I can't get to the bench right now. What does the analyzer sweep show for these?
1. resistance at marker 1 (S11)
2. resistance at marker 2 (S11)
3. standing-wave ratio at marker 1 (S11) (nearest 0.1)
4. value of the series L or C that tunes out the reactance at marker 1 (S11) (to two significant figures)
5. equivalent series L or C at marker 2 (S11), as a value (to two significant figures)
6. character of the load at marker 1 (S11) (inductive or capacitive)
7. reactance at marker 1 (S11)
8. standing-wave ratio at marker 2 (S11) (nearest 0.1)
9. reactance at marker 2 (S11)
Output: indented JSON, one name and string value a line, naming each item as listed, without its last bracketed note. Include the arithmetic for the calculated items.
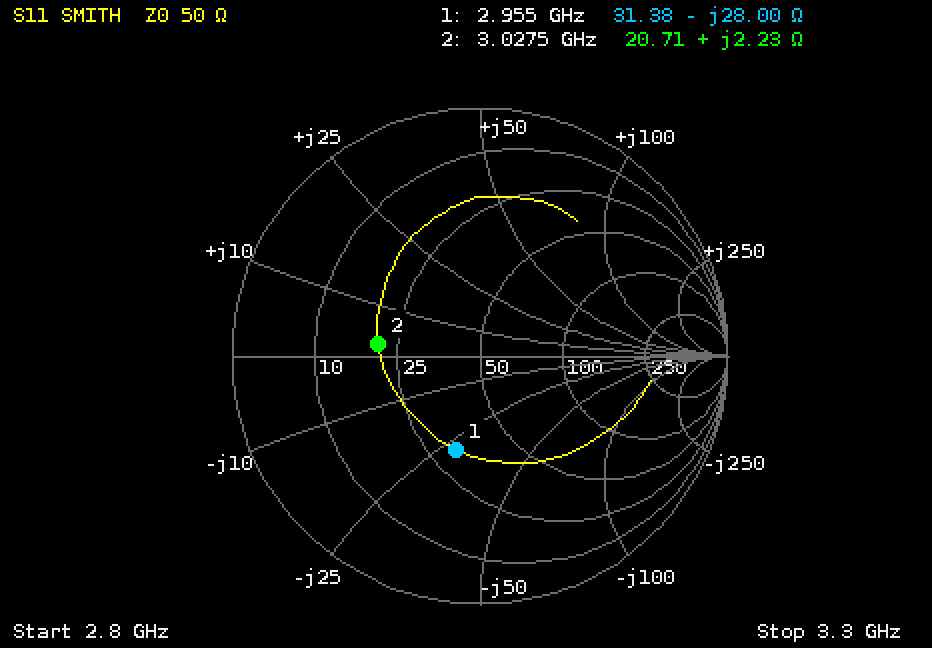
{
  "resistance at marker 1": "31.38 Ω",
  "resistance at marker 2": "20.71 Ω",
  "standing-wave ratio at marker 1 (S11)": "2.3",
  "value of the series L or C that tunes out the reactance at marker 1 (S11)": "L = 28 Ω/(2π × 2.955 GHz) ≈ 1.5 nH",
  "equivalent series L or C at marker 2 (S11), as a value": "L = 2.23 Ω/(2π × 3.0275 GHz) ≈ 117 pH, so 120 pH to two significant figures",
  "character of the load at marker 1 (S11)": "capacitive",
  "reactance at marker 1": "-28.00 Ω",
  "standing-wave ratio at marker 2 (S11)": "2.4",
  "reactance at marker 2": "+2.23 Ω"
}
